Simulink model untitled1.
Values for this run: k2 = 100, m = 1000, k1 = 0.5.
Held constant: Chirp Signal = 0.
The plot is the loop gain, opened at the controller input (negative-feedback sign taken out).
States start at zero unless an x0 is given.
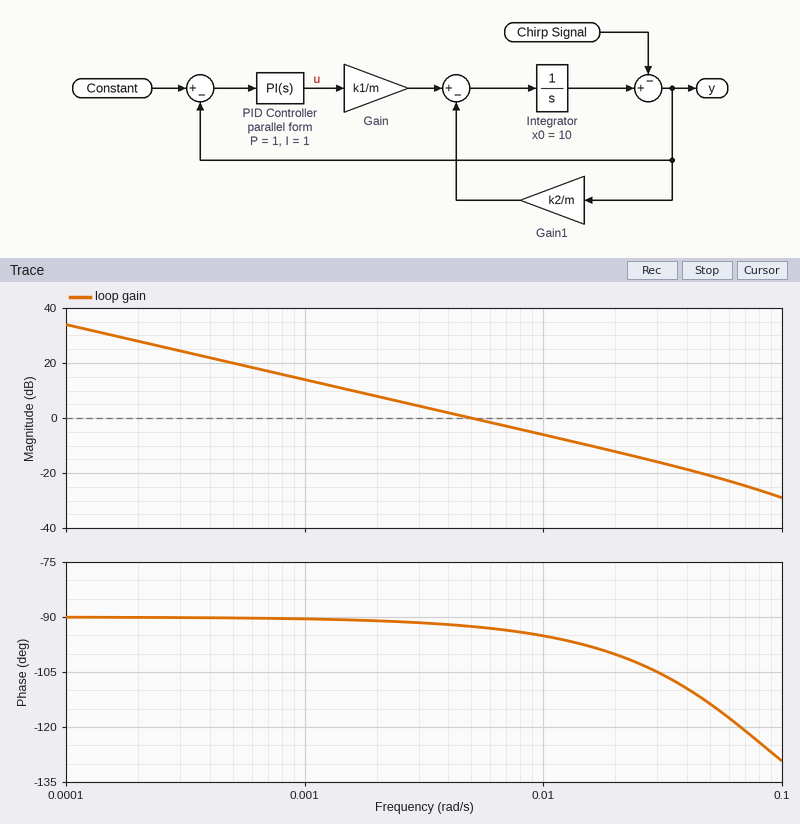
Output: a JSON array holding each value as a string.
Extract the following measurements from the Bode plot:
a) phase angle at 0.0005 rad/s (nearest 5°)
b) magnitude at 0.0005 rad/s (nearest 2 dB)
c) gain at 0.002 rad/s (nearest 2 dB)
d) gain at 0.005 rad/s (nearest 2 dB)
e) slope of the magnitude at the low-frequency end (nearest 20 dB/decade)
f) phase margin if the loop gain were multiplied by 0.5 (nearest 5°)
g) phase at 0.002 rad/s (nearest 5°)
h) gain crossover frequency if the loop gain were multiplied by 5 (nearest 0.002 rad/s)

["-90°", "20 dB", "8 dB", "0 dB", "-20 dB/decade", "90°", "-90°", "0.024 rad/s"]
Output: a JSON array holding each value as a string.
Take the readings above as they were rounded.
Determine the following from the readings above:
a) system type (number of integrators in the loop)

["1"]
